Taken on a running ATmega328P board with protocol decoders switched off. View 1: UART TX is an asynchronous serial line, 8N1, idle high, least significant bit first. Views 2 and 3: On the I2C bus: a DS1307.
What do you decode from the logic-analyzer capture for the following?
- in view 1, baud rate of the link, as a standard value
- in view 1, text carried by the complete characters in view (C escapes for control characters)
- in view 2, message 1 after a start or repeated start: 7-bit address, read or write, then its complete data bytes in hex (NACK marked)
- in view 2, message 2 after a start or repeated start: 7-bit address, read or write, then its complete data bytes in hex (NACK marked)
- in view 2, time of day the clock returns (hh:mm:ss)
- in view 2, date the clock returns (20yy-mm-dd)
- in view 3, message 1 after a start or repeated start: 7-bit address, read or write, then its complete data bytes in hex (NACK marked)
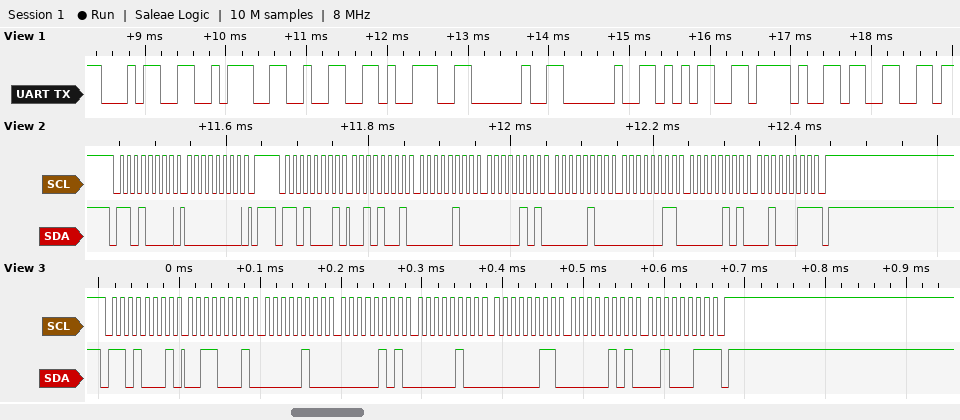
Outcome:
9600 baud
"4:29  5/3"
0x68 write: 00
0x68 read: 29 04 05 04 03 05 23 NACK
05:04:29
2023-05-03
0x68 read: 31 04 05 04 03 05 23 NACK
